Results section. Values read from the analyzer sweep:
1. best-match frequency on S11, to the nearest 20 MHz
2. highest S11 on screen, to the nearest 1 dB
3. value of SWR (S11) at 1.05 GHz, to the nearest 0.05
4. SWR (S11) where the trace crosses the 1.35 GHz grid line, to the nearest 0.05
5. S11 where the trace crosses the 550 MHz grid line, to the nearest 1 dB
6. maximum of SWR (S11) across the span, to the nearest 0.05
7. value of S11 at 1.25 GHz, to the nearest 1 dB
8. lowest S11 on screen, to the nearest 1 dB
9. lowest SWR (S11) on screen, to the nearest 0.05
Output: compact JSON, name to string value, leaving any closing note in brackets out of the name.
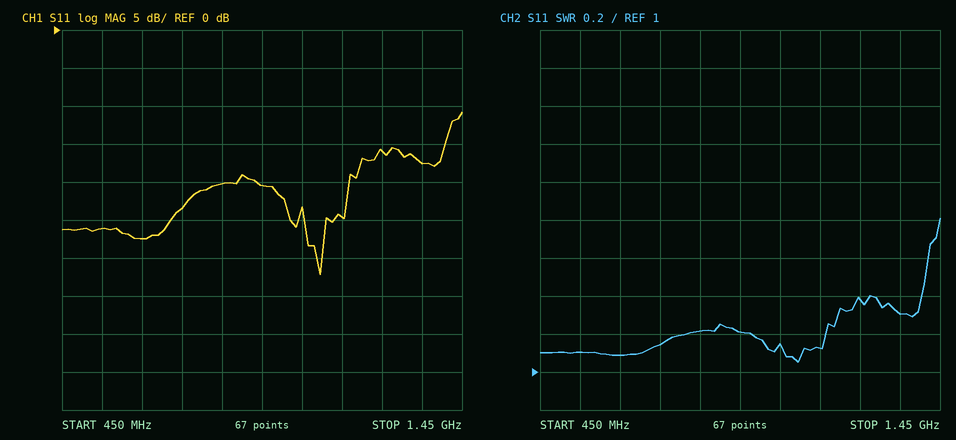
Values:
{"best-match frequency on S11, to the nearest 20 MHz": "1.10 GHz", "highest S11 on screen, to the nearest 1 dB": "-11 dB", "value of SWR (S11) at 1.05 GHz, to the nearest 0.05": "1.15", "SWR (S11) where the trace crosses the 1.35 GHz grid line, to the nearest 0.05": "1.30", "S11 where the trace crosses the 550 MHz grid line, to the nearest 1 dB": "-26 dB", "maximum of SWR (S11) across the span, to the nearest 0.05": "1.80", "value of S11 at 1.25 GHz, to the nearest 1 dB": "-16 dB", "lowest S11 on screen, to the nearest 1 dB": "-32 dB", "lowest SWR (S11) on screen, to the nearest 0.05": "1.05"}
